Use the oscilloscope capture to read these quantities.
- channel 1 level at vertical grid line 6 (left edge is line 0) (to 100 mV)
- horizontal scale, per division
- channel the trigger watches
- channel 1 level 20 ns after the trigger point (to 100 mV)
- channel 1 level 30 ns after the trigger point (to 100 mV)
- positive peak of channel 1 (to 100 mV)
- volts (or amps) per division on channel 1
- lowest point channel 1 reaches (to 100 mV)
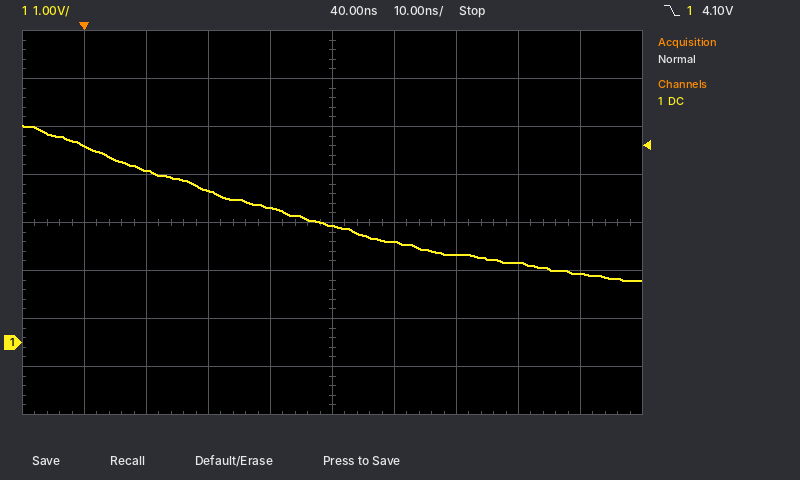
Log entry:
2.1 V
10 ns
channel 1
3.2 V
2.8 V
4.5 V
1 V
1.3 V
